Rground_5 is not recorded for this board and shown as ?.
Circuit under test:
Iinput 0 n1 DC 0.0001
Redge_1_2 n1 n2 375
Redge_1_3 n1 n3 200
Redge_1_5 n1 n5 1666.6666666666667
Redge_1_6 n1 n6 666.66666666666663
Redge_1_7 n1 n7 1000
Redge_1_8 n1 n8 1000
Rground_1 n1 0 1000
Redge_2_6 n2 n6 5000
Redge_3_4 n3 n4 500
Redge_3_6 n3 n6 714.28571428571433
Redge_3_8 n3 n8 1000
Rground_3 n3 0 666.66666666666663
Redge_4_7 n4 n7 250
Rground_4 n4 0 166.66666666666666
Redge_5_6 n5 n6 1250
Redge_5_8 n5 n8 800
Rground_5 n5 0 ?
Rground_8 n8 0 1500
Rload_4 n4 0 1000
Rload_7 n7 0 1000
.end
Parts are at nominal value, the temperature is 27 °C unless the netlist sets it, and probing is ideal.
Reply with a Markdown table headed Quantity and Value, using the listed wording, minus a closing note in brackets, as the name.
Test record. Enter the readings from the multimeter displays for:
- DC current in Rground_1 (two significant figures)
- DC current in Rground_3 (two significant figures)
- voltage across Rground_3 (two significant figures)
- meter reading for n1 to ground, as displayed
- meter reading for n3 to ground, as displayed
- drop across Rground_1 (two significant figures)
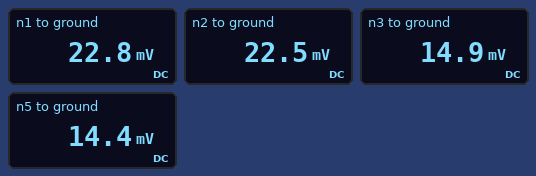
| Quantity | Value |
|---|---|
| DC current in Rground_1 | 23 µA |
| DC current in Rground_3 | 22 µA |
| voltage across Rground_3 | 15 mV |
| meter reading for n1 to ground, as displayed | 22.8 mV |
| meter reading for n3 to ground, as displayed | 14.9 mV |
| drop across Rground_1 | 23 mV |
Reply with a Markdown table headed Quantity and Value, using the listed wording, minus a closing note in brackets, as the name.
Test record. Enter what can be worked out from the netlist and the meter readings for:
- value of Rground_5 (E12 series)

| Quantity | Value |
|---|---|
| value of Rground_5 | 1.8 kΩ |
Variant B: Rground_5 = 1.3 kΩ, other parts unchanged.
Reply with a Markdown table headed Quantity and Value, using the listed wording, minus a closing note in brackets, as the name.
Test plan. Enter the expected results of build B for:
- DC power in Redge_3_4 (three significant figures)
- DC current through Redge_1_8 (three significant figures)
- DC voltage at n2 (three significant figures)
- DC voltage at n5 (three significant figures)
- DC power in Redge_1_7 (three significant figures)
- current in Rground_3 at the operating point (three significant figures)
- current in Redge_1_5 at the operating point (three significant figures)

| Quantity | Value |
|---|---|
| DC power in Redge_3_4 | 213 nW |
| DC current through Redge_1_8 | 8.82 µA |
| DC voltage at n2 | 22.1 mV |
| DC voltage at n5 | 13.1 mV |
| DC power in Redge_1_7 | 251 nW |
| current in Rground_3 at the operating point | 21.9 µA |
| current in Redge_1_5 at the operating point | 5.63 µA |
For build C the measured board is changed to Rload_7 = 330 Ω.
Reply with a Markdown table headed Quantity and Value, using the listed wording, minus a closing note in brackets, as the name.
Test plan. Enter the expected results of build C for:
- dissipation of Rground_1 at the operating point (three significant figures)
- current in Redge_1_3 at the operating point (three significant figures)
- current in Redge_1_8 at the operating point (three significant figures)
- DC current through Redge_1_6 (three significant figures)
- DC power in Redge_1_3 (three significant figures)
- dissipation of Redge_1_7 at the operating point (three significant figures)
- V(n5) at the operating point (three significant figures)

| Quantity | Value |
|---|---|
| dissipation of Rground_1 at the operating point | 494 nW |
| current in Redge_1_3 at the operating point | 39.1 µA |
| current in Redge_1_8 at the operating point | 8.42 µA |
| DC current through Redge_1_6 | 6.78 µA |
| DC power in Redge_1_3 | 306 nW |
| dissipation of Redge_1_7 at the operating point | 312 nW |
| V(n5) at the operating point | 14.0 mV |
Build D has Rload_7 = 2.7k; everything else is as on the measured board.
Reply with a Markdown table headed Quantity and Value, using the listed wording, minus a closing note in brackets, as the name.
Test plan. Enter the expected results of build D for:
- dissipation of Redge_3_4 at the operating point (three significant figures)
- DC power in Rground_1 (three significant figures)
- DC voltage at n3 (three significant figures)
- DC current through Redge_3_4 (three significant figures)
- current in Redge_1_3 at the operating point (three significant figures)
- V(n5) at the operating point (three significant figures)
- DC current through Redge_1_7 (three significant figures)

| Quantity | Value |
|---|---|
| dissipation of Redge_3_4 at the operating point | 219 nW |
| DC power in Rground_1 | 537 nW |
| DC voltage at n3 | 15.2 mV |
| DC current through Redge_3_4 | 20.9 µA |
| current in Redge_1_3 at the operating point | 39.8 µA |
| V(n5) at the operating point | 14.6 mV |
| DC current through Redge_1_7 | 15.3 µA |
